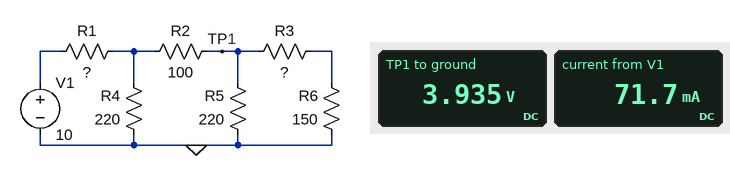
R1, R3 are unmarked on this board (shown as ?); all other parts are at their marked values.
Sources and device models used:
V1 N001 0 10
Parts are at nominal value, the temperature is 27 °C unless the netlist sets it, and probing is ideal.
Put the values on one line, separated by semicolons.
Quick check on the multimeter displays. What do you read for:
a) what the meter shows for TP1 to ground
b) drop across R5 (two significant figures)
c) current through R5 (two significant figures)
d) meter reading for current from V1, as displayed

3.935 V; 3.9 V; 18 mA; 71.7 mA
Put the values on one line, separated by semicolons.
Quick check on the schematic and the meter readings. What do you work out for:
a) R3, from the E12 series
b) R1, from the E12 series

56 Ω; 33 Ω
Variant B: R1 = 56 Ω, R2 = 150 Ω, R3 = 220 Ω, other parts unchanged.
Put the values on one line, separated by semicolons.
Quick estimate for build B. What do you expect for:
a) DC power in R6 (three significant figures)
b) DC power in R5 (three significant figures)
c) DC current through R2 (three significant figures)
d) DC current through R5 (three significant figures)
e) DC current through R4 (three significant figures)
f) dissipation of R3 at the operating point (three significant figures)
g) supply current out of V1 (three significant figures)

12.0 mW; 49.7 mW; 24.0 mA; 15.0 mA; 31.4 mA; 17.6 mW; 55.3 mA
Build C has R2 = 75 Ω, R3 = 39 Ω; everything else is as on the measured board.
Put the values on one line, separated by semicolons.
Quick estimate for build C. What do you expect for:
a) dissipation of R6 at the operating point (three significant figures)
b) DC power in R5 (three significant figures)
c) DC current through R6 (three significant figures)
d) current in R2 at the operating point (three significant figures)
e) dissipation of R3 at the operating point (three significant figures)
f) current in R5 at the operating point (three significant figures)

77.8 mW; 84.2 mW; 22.8 mA; 42.3 mA; 20.2 mW; 19.6 mA
